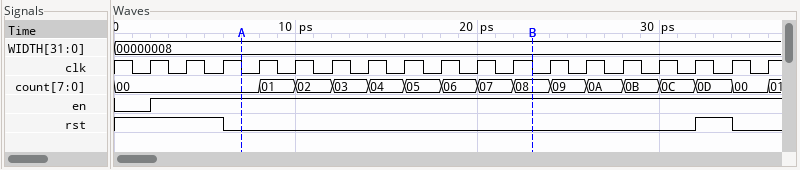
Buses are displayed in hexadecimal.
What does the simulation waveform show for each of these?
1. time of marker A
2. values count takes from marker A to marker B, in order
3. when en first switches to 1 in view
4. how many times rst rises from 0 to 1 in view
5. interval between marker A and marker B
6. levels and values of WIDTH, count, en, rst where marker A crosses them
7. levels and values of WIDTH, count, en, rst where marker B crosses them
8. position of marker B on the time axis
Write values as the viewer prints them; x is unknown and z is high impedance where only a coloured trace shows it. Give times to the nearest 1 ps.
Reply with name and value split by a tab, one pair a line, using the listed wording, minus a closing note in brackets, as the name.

time of marker A	7 ps
values count takes from marker A to marker B, in order	00, 01, 02, 03, 04, 05, 06, 07, 08
when en first switches to 1 in view	2 ps
how many times rst rises from 0 to 1 in view	1
interval between marker A and marker B	16 ps
levels and values of WIDTH, count, en, rst where marker A crosses them	WIDTH=00000008, count=00, en=1, rst=0
levels and values of WIDTH, count, en, rst where marker B crosses them	WIDTH=00000008, count=08, en=1, rst=0
position of marker B on the time axis	23 ps
